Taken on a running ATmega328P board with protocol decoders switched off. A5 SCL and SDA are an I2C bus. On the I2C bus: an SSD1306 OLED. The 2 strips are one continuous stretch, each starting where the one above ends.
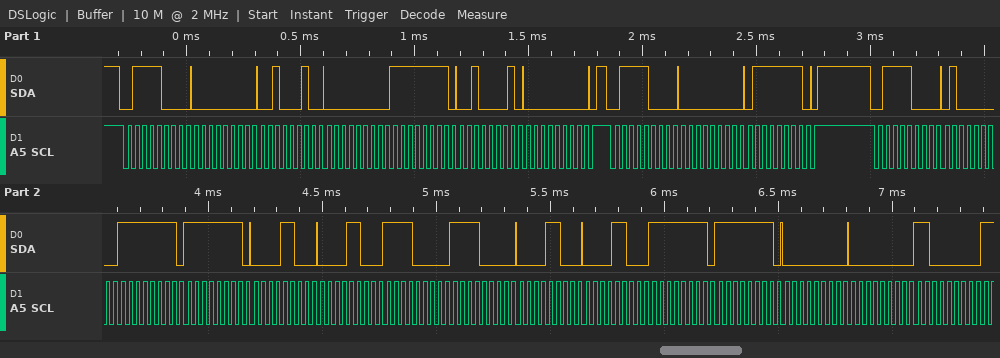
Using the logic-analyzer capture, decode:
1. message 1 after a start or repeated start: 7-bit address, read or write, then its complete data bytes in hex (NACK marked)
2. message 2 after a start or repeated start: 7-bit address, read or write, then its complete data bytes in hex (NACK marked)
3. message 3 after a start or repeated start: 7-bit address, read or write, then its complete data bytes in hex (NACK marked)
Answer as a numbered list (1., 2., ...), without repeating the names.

1. 0x3C write: 00 22 00 FF 21 00
2. 0x3C write: 00 7F
3. 0x3C write: 40 FF FF 0C 0C F0 F0 0C 0C FF FF 00 00 C0
